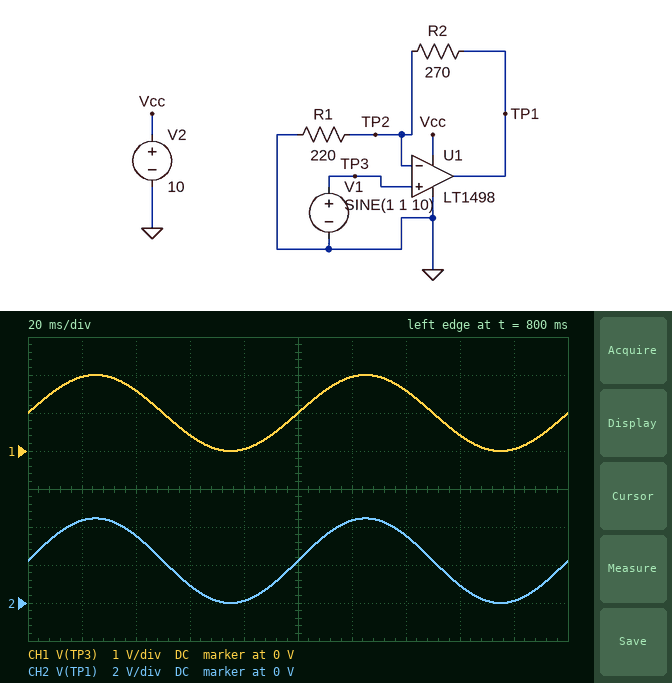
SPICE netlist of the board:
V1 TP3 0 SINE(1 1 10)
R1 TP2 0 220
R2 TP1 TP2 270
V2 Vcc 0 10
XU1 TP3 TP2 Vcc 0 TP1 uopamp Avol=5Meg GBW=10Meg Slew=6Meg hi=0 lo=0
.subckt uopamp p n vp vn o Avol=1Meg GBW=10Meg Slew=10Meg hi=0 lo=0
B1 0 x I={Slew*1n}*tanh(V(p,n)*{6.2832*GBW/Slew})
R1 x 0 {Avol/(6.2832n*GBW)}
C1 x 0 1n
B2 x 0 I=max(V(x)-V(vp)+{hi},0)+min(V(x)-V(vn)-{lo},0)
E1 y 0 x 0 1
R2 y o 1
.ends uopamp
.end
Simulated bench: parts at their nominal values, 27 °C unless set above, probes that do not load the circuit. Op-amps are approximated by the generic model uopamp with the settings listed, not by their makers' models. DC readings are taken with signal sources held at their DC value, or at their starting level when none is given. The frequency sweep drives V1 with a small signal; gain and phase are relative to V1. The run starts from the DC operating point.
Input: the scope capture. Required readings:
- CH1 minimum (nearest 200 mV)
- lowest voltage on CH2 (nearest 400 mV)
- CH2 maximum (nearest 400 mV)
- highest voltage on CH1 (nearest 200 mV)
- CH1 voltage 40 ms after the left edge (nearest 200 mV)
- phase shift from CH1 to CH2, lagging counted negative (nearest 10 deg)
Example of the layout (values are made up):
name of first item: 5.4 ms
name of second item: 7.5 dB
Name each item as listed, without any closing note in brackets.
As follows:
CH1 minimum: 0 V
lowest voltage on CH2: 0 V
CH2 maximum: 4.4 V
highest voltage on CH1: 2.0 V
CH1 voltage 40 ms after the left edge: 1.6 V
phase shift from CH1 to CH2, lagging counted negative: 0 deg
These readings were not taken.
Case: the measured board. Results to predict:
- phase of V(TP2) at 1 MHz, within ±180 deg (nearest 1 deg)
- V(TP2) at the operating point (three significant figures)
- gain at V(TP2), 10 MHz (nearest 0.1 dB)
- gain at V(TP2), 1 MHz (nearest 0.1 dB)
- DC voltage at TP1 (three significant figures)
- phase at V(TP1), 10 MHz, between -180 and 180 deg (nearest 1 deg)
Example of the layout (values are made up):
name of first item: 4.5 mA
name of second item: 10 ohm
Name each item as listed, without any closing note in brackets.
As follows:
phase of V(TP2) at 1 MHz, within ±180 deg: -13 deg
V(TP2) at the operating point: 1.00 V
gain at V(TP2), 10 MHz: -7.8 dB
gain at V(TP2), 1 MHz: -0.2 dB
DC voltage at TP1: 2.23 V
phase at V(TP1), 10 MHz, between -180 and 180 deg: -66 deg
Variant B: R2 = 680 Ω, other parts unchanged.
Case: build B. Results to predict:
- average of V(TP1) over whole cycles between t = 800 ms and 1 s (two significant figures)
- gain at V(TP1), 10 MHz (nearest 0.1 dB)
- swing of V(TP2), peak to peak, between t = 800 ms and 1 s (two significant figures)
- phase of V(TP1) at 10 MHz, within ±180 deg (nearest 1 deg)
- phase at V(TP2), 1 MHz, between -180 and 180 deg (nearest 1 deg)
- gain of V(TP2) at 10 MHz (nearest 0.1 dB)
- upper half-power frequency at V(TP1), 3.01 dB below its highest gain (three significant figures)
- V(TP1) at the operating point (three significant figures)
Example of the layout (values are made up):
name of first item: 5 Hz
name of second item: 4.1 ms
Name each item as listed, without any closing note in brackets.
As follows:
average of V(TP1) over whole cycles between t = 800 ms and 1 s: 4.1 V
gain at V(TP1), 10 MHz: -0.3 dB
swing of V(TP2), peak to peak, between t = 800 ms and 1 s: 2.0 V
phase of V(TP1) at 10 MHz, within ±180 deg: -76 deg
phase at V(TP2), 1 MHz, between -180 and 180 deg: -22 deg
gain of V(TP2) at 10 MHz: -12.5 dB
upper half-power frequency at V(TP1), 3.01 dB below its highest gain: 2.44 MHz
V(TP1) at the operating point: 4.09 V
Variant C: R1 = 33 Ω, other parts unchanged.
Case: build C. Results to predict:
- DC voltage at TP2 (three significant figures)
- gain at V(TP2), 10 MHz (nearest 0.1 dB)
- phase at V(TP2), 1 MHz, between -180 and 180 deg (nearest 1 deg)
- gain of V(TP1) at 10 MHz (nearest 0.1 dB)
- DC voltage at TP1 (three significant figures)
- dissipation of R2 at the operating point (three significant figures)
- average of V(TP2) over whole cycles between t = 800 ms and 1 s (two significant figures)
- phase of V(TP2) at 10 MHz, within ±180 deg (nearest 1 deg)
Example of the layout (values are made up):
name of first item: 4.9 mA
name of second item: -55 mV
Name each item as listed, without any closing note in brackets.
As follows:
DC voltage at TP2: 1.00 V
gain at V(TP2), 10 MHz: -19.3 dB
phase at V(TP2), 1 MHz, between -180 and 180 deg: -43 deg
gain of V(TP1) at 10 MHz: -0.1 dB
DC voltage at TP1: 9.18 V
dissipation of R2 at the operating point: 248 mW
average of V(TP2) over whole cycles between t = 800 ms and 1 s: 720 mV
phase of V(TP2) at 10 MHz, within ±180 deg: -84 deg
